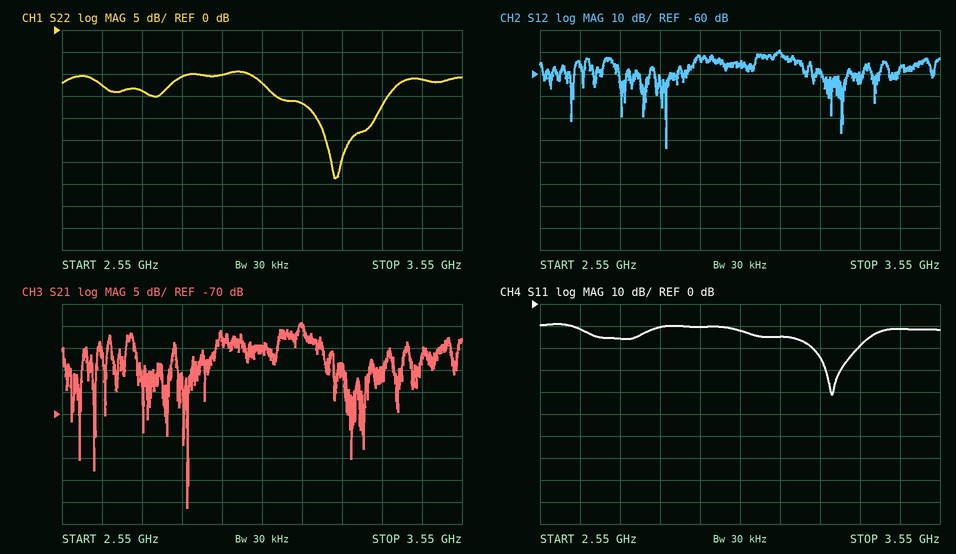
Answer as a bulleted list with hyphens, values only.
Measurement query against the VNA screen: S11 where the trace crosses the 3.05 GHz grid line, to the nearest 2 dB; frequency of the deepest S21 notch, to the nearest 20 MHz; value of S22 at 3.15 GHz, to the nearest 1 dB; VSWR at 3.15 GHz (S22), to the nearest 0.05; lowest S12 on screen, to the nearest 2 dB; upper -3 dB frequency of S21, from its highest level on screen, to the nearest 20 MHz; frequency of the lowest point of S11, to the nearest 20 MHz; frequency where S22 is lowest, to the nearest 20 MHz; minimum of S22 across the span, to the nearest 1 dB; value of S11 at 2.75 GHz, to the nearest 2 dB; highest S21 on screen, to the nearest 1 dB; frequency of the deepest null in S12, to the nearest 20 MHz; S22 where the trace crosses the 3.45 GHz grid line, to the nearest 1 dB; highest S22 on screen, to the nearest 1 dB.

- -12 dB
- 2.86 GHz
- -17 dB
- 1.35
- -94 dB
- 3.16 GHz
- 3.28 GHz
- 3.24 GHz
- -34 dB
- -16 dB
- -49 dB
- 2.86 GHz
- -11 dB
- -9 dB
